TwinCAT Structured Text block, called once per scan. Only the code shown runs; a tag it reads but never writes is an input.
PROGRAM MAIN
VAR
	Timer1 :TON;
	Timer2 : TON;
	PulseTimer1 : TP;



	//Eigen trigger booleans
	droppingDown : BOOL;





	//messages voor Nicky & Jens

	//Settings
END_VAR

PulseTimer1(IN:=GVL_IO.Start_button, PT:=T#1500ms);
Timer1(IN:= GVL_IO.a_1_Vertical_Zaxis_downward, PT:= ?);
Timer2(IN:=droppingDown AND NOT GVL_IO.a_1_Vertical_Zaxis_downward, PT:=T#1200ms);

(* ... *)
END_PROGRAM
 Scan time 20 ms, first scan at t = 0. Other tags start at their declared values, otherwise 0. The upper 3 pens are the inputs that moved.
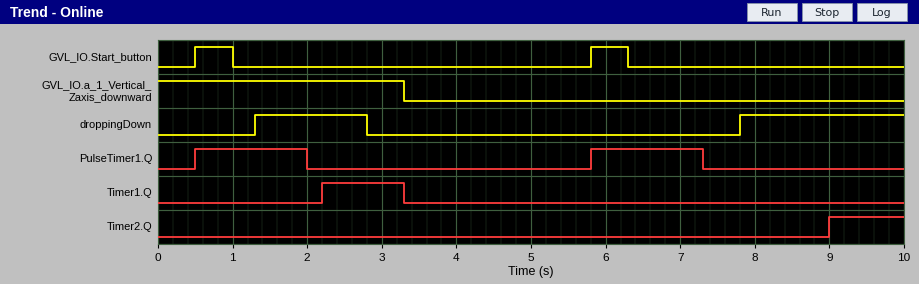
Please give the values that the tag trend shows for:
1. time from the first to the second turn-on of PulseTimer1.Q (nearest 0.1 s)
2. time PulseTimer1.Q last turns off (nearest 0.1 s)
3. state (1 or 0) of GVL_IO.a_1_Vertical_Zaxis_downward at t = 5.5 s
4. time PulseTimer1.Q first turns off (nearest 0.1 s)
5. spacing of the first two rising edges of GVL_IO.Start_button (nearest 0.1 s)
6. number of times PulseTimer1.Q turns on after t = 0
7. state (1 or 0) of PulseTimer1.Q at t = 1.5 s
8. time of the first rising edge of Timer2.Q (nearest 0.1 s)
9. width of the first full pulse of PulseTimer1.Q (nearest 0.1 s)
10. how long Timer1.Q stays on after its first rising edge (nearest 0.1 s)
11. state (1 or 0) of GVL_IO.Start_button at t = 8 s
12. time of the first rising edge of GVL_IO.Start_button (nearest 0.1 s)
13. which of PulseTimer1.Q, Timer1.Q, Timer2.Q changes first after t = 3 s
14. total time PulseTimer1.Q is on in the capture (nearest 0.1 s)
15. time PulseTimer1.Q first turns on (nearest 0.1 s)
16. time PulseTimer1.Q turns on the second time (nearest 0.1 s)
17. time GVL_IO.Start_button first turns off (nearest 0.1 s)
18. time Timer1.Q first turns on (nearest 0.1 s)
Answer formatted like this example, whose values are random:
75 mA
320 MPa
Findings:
5.3 s
7.3 s
0
2.0 s
5.3 s
2
1
9.0 s
1.5 s
1.1 s
0
0.5 s
Timer1.Q
3.0 s
0.5 s
5.8 s
1.0 s
2.2 s
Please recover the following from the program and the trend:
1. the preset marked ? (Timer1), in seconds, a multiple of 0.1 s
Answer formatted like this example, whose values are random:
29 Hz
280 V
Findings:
2.2 s
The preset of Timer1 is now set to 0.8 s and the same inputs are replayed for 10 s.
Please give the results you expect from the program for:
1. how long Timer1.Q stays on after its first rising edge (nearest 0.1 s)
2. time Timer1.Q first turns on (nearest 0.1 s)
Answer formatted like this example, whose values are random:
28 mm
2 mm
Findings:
2.5 s
0.8 s
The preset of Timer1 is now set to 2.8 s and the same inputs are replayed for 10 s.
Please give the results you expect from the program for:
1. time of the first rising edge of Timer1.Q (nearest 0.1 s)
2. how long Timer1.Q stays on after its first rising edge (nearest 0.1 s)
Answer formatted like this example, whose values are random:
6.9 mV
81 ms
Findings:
2.8 s
0.5 s
